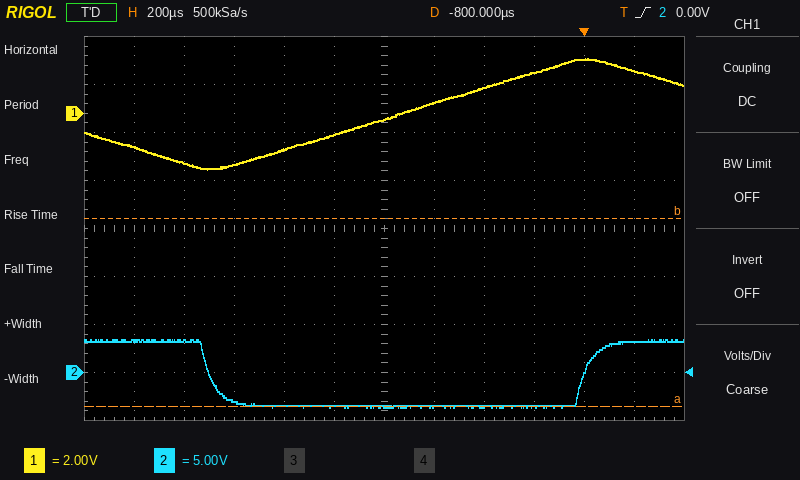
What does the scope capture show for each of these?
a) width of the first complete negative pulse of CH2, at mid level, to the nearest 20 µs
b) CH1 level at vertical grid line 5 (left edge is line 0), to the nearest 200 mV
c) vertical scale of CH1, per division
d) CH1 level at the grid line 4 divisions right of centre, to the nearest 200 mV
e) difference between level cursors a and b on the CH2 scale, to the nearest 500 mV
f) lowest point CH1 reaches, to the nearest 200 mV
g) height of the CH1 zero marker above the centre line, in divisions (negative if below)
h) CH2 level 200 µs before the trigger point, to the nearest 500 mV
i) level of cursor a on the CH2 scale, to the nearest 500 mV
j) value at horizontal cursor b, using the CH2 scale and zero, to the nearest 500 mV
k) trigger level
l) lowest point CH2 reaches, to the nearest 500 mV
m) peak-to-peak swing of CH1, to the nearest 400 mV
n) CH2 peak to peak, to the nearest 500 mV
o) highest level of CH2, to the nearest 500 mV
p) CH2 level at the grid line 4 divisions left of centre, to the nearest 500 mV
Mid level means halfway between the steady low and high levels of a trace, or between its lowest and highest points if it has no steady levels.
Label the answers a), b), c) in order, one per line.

a) 1.50 ms
b) -800 mV
c) 2 V
d) 2.2 V
e) 19.5 V
f) -2.4 V
g) +2.4 div
h) -3.5 V
i) -3.5 V
j) 16.0 V
k) 0.00 V
l) -3.5 V
m) 4.8 V
n) 7.0 V
o) 3.5 V
p) 3.5 V
